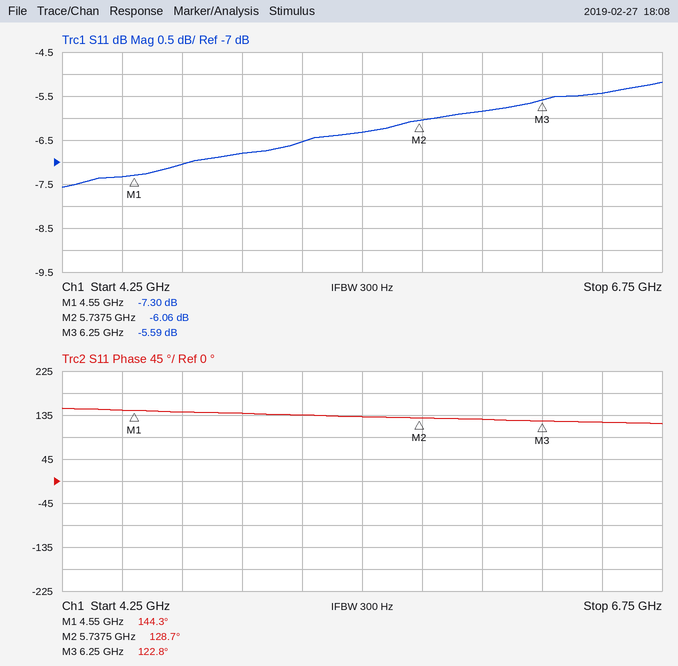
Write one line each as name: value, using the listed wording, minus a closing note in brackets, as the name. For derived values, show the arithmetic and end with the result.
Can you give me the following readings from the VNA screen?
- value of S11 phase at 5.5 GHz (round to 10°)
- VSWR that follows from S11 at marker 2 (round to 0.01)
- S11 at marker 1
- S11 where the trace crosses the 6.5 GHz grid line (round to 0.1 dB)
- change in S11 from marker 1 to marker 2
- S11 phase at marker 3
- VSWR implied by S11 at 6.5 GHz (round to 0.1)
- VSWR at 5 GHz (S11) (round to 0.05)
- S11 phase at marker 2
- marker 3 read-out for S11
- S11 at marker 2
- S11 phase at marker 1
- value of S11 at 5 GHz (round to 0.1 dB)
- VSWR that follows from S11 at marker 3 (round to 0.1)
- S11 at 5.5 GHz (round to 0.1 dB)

value of S11 phase at 5.5 GHz: 130°
VSWR that follows from S11 at marker 2: (1 + 0.4977)/(1 − 0.4977) ≈ 2.98
S11 at marker 1: -7.30 dB
S11 where the trace crosses the 6.5 GHz grid line: -5.4 dB
change in S11 from marker 1 to marker 2: -6.06 − (-7.3) = 1.24 dB
S11 phase at marker 3: 122.8°
VSWR implied by S11 at 6.5 GHz: |Γ| = 10^(-5.4/20) = 0.5370; VSWR = (1 + 0.5370)/(1 − 0.5370) ≈ 3.3
VSWR at 5 GHz (S11): |Γ| = 10^(-6.8/20) = 0.4571; VSWR = (1 + 0.4571)/(1 − 0.4571) ≈ 2.68, so 2.70 to the nearest 0.05
S11 phase at marker 2: 128.7°
marker 3 read-out for S11: -5.59 dB
S11 at marker 2: -6.06 dB
S11 phase at marker 1: 144.3°
value of S11 at 5 GHz: -6.8 dB
VSWR that follows from S11 at marker 3: (1 + 0.5254)/(1 − 0.5254) ≈ 3.2
S11 at 5.5 GHz: -6.3 dB
